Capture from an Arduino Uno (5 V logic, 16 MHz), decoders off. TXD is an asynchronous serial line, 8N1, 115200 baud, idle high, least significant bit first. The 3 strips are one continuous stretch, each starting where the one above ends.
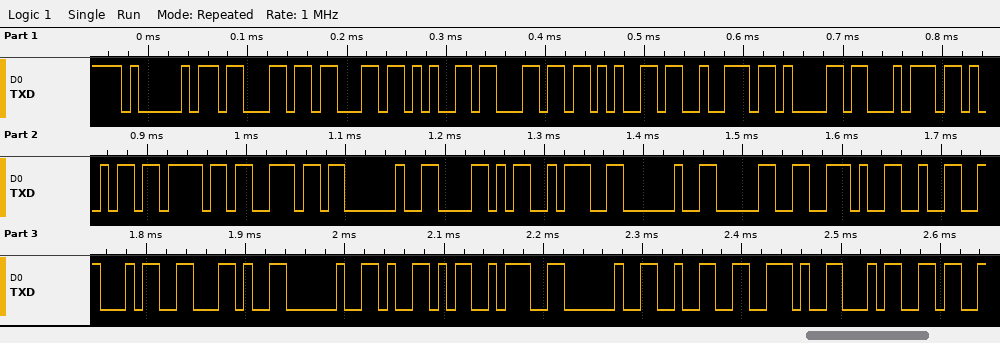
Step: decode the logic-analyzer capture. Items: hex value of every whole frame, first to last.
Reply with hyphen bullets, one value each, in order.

- 0x41 0x63 0x63 0x65 0x6C 0x65 0x72 0x61 0x74 0x69 0x6F 0x6E 0x20 0x58 0x3A 0x20 0x30 0x2E 0x32 0x34 0x2C 0x20 0x59 0x3A 0x20 0x32 0x2E 0x34
